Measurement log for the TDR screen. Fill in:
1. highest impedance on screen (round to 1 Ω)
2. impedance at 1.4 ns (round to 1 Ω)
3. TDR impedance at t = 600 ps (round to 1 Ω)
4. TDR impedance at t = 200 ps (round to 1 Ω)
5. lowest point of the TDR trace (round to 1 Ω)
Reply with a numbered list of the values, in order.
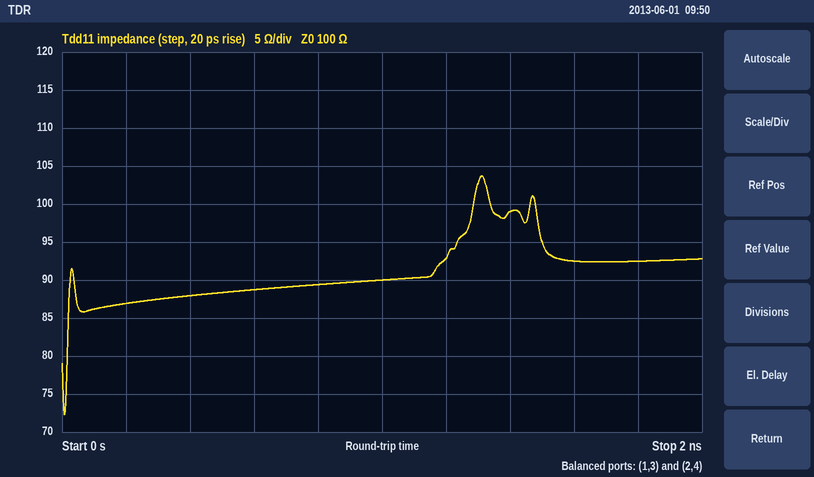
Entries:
1. 104 Ω
2. 99 Ω
3. 89 Ω
4. 87 Ω
5. 72 Ω
